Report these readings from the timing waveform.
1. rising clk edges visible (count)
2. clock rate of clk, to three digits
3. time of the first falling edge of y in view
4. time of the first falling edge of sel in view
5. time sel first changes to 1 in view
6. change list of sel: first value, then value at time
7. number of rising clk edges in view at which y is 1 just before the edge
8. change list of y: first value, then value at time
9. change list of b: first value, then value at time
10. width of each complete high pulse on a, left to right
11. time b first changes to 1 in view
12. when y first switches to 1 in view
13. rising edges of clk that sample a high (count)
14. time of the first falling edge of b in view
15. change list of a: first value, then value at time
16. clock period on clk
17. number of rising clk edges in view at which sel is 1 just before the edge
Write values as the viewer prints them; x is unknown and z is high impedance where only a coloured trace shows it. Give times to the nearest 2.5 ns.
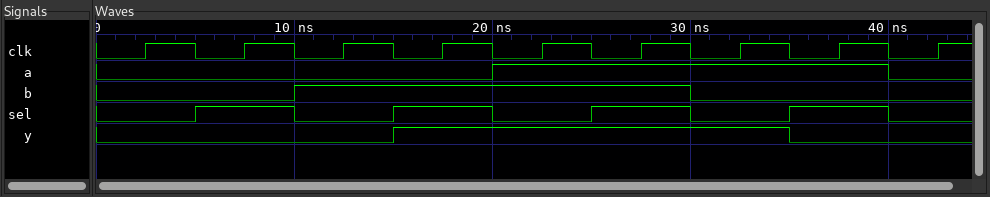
9
200 MHz
35 ns
10 ns
5 ns
0, 1 at 5 ns, 0 at 10 ns, 1 at 15 ns, 0 at 20 ns, 1 at 25 ns, 0 at 30 ns, 1 at 35 ns, 0 at 40 ns
4
0, 1 at 15 ns, 0 at 35 ns
0, 1 at 10 ns, 0 at 30 ns
20 ns
10 ns
15 ns
4
30 ns
0, 1 at 20 ns, 0 at 40 ns
5 ns
4
